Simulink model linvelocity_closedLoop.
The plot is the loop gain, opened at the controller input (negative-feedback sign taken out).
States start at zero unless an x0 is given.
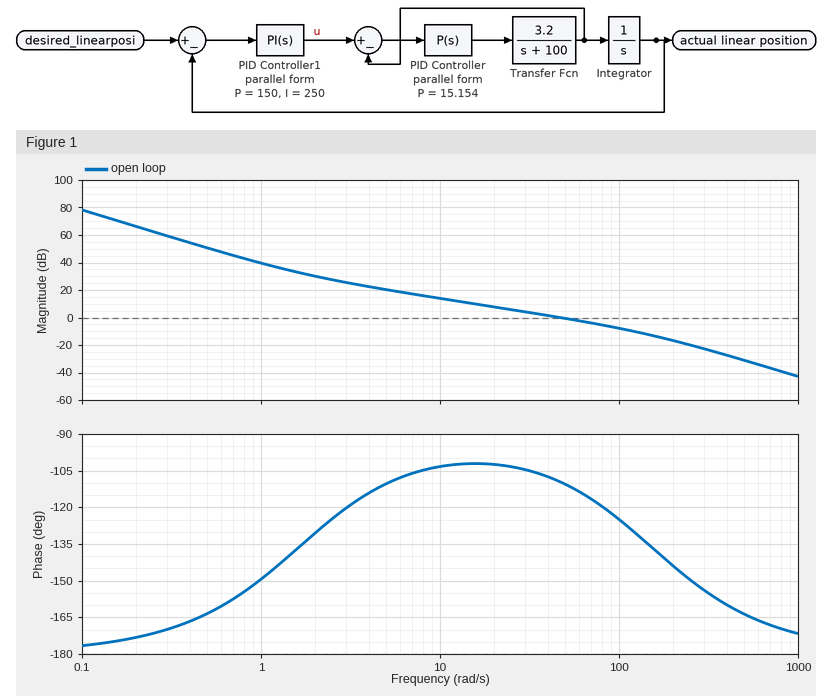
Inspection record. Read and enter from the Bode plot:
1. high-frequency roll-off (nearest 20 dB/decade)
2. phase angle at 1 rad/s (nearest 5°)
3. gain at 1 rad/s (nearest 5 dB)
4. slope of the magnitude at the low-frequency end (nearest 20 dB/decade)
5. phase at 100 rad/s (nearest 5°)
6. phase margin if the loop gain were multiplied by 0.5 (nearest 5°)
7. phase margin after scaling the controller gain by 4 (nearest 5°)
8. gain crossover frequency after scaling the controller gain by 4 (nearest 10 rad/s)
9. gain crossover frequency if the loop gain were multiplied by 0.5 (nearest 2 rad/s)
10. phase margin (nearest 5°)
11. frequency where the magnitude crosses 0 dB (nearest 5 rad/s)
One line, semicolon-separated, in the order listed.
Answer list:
-40 dB/decade; -150°; 40 dB; -40 dB/decade; -125°; 75°; 45°; 140 rad/s; 24 rad/s; 70°; 45 rad/s
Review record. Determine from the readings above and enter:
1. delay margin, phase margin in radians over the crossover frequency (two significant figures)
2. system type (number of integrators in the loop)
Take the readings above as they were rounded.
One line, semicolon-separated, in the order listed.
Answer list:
0.027 s; 2
